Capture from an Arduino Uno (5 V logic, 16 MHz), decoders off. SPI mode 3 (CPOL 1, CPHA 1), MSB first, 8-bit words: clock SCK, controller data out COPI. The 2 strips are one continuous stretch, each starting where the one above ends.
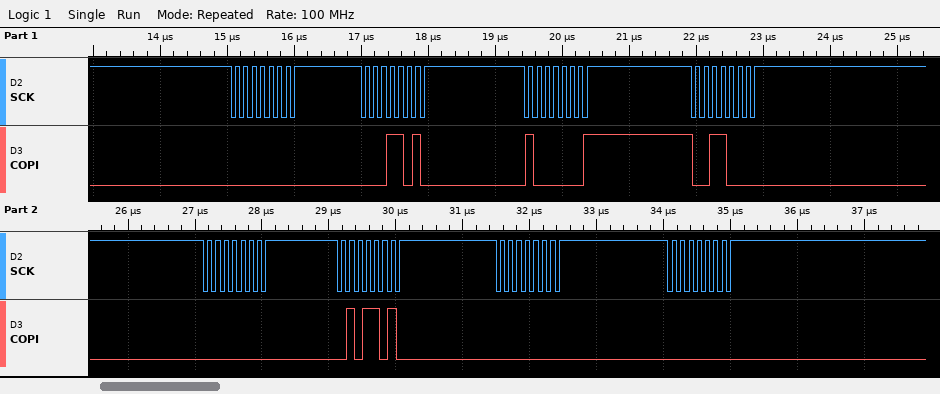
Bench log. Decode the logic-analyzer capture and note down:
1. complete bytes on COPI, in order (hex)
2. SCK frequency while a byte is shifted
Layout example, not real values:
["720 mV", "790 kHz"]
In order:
["00 1A 81 30 00 5A 00 00", "8 MHz"]
